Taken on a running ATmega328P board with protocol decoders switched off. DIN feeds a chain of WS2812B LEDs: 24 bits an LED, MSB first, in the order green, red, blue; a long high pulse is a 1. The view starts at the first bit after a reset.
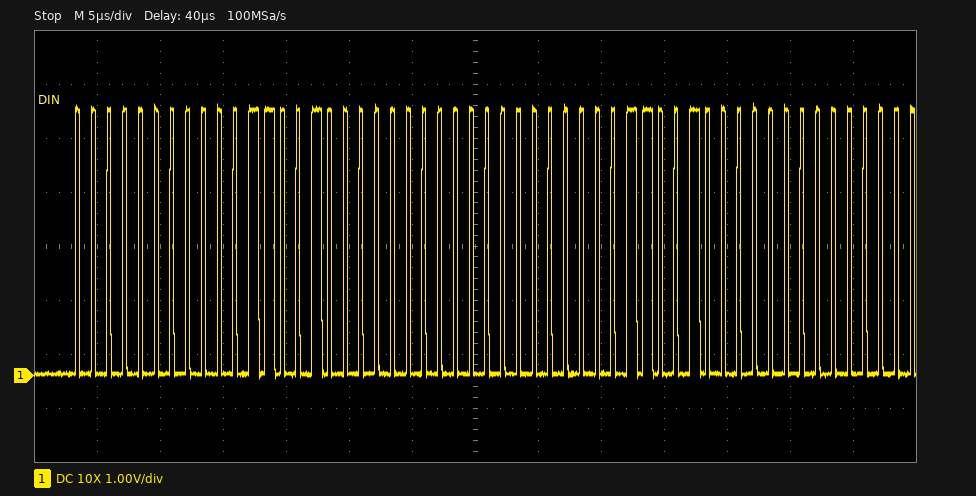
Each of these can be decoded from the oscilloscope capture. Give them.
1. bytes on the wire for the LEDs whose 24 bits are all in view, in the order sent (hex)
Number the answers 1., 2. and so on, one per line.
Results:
1. 00 19 00 00 19 00
